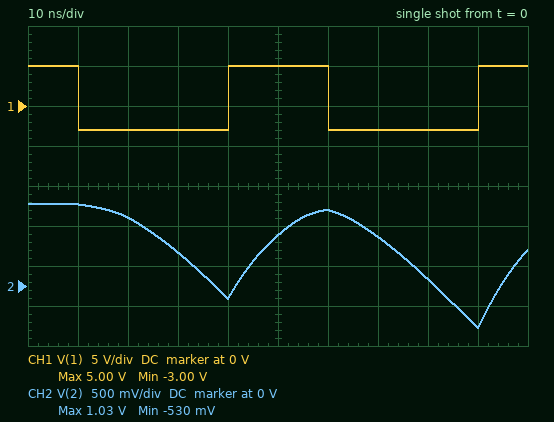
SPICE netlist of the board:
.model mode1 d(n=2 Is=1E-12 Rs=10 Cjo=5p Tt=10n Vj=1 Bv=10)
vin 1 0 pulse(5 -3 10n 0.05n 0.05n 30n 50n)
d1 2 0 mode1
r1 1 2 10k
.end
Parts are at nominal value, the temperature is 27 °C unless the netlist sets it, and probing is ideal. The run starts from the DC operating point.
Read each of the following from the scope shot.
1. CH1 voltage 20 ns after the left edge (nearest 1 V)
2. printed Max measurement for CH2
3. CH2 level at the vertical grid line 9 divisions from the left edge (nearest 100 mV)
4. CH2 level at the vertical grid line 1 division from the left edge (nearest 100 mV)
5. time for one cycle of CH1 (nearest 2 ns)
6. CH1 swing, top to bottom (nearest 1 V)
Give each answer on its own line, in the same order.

-3 V
1.03 V
-500 mV
1.0 V
50 ns
8 V
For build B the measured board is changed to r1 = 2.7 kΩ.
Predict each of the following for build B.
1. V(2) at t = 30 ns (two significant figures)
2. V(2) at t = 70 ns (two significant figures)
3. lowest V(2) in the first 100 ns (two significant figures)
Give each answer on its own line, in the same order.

-1.5 V
190 mV
-2.7 V
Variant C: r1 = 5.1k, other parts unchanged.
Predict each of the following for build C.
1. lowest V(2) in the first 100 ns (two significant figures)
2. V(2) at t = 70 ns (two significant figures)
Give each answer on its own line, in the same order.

-1.7 V
470 mV
